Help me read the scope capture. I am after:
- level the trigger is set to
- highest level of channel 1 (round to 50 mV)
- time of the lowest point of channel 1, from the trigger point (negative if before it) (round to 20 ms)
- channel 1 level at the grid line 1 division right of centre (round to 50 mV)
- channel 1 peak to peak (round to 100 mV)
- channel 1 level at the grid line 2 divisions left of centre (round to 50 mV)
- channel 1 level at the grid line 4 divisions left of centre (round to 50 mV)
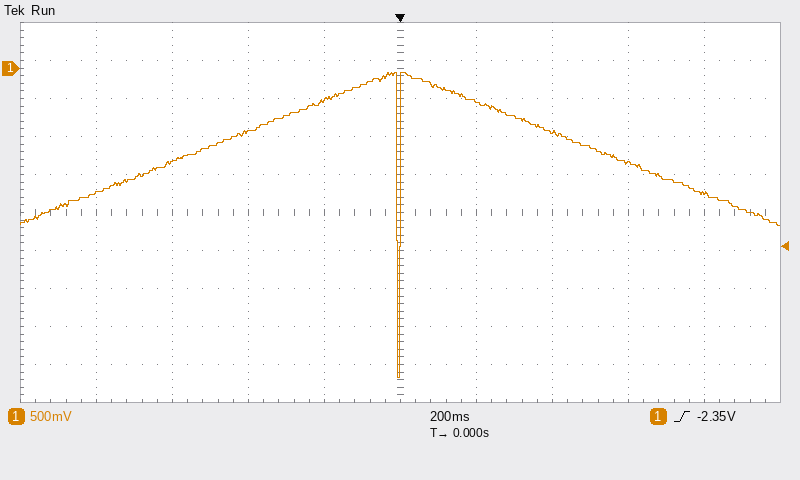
-2.35 V
-50 mV
0 ms
-450 mV
4.00 V
-850 mV
-1.65 V
